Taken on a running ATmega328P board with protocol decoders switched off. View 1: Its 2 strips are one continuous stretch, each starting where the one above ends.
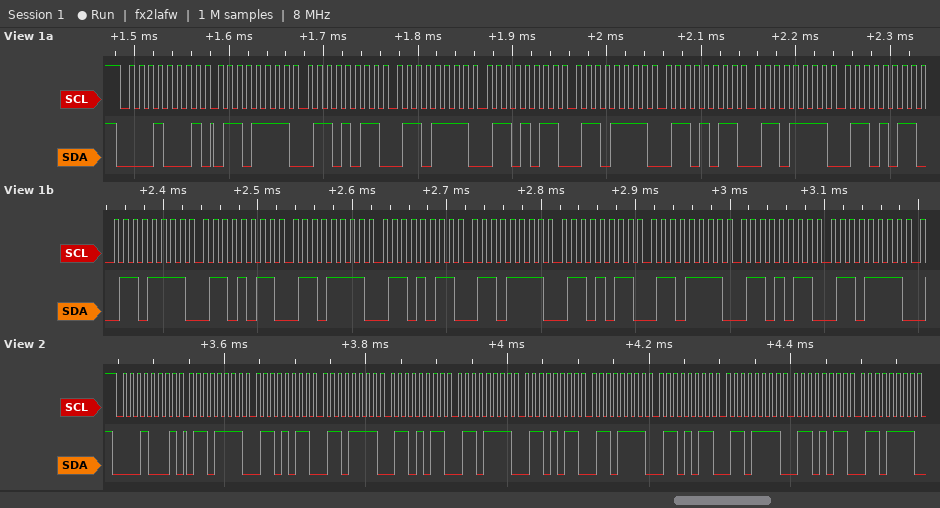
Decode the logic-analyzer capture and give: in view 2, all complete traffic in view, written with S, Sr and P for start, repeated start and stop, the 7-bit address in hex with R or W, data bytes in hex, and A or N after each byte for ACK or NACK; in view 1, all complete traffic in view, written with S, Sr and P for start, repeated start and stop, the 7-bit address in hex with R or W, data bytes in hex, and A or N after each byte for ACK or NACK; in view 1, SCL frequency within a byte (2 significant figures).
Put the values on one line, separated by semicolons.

S 08R A 6F A 6B A 6F A 6B A 6F A 6B A 6F A 6B A 6F A 6B A 6F A; S 08R A 6F A 6B A 6F A 6B A 6F A 6B A 6F A 6B A 6F A 6B A 6F A 6B A 6F A 6B A 6F A 6B A 6F A; 100 kHz
